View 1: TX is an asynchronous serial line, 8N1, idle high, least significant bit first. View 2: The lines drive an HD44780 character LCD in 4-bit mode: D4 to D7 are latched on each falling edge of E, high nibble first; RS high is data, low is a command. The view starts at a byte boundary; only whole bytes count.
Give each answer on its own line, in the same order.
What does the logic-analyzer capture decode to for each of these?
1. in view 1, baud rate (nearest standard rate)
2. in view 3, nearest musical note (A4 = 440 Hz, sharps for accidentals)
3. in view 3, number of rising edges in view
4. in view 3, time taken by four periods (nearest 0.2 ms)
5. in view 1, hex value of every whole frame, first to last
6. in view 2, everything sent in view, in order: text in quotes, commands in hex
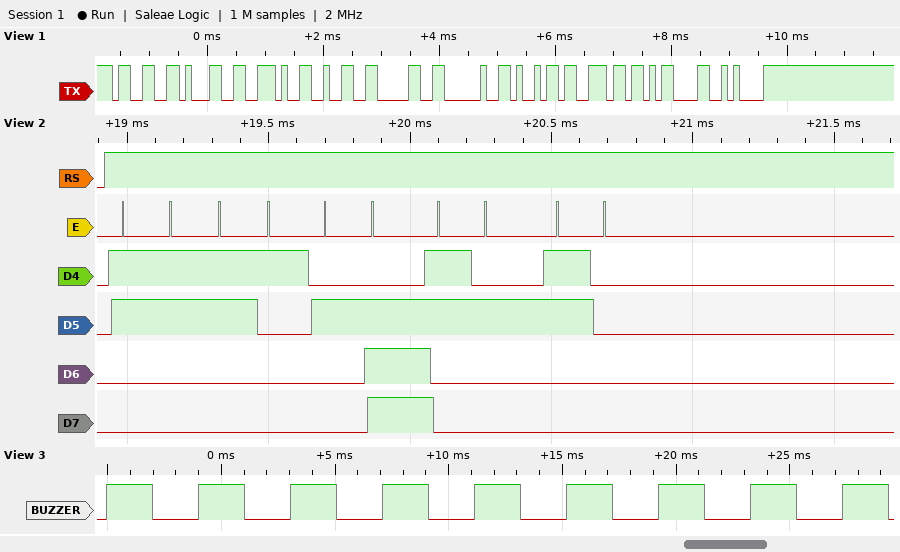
9600 baud
B3
9
16.2 ms
33 31 2E 32 30 20 69 6E 0D 0A
"31.20"
